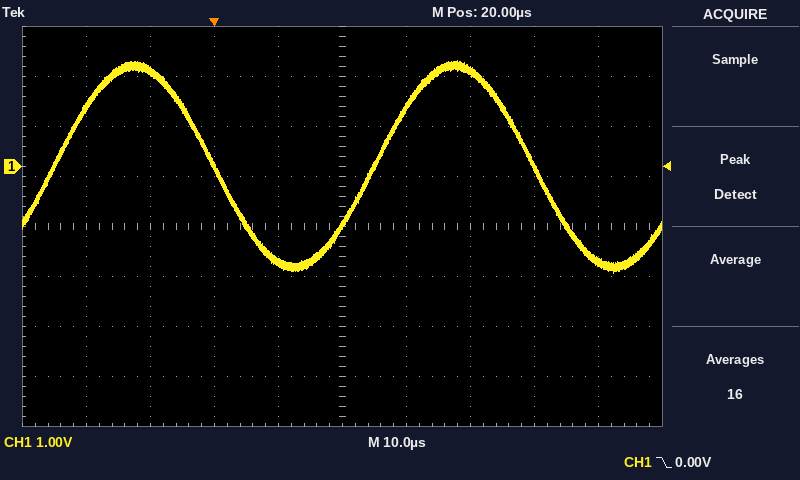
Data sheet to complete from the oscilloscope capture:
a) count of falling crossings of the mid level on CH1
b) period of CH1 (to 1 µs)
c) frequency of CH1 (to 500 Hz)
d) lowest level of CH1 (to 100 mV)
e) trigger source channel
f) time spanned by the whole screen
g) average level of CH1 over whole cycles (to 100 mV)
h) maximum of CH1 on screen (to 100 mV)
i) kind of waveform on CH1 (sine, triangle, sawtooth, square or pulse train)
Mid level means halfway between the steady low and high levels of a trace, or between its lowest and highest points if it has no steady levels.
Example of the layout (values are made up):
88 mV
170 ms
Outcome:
2
50 µs
20.0 kHz
-2.1 V
CH1
100 µs
0.0 V
2.1 V
sine
